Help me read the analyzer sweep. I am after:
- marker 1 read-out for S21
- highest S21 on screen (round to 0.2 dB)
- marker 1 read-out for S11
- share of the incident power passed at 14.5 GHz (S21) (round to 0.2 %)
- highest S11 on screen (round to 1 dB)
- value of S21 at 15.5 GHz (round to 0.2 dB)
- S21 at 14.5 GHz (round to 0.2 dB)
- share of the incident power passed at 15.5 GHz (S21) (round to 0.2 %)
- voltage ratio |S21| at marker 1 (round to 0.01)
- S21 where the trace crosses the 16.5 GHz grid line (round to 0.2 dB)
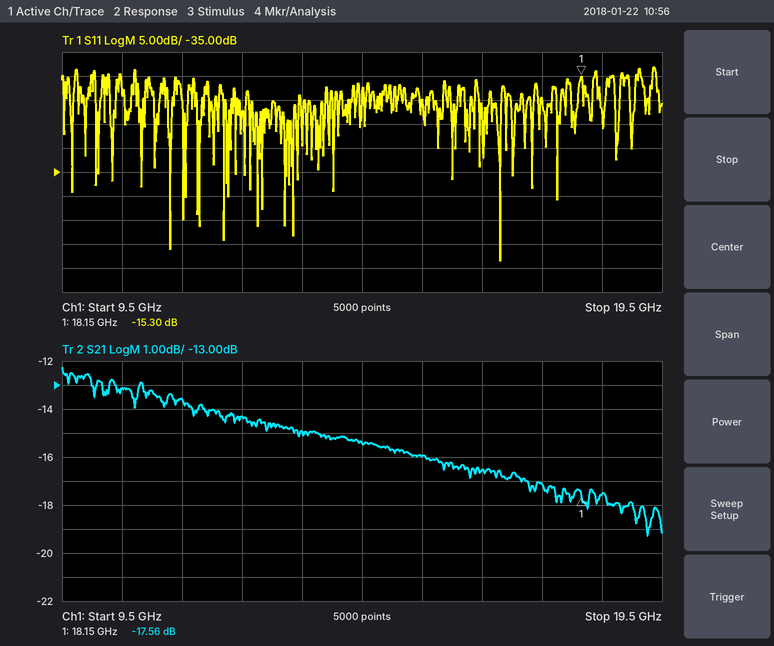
-17.56 dB
-12.2 dB
-15.30 dB
2.8 %
-13 dB
-16.0 dB
-15.4 dB
2.6 %
0.13
-16.6 dB
